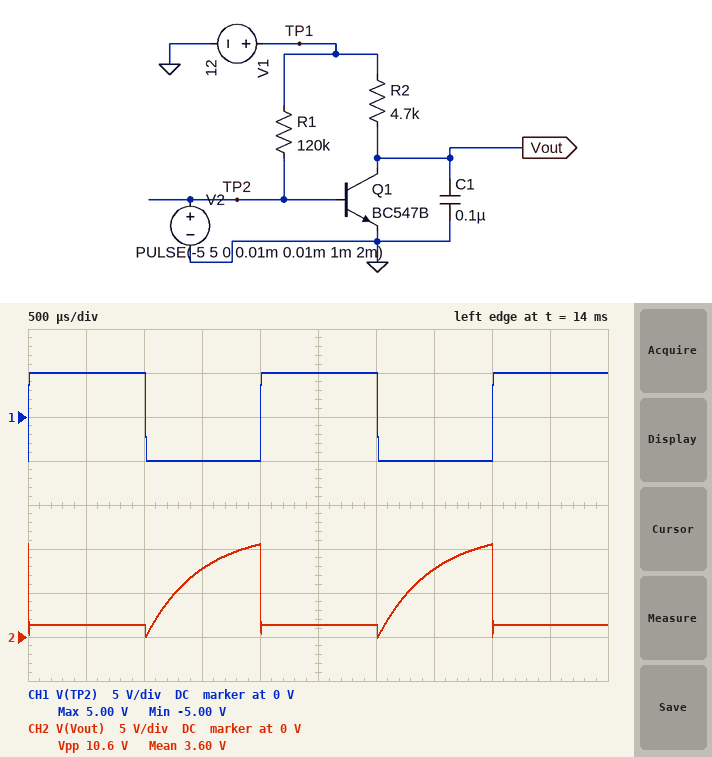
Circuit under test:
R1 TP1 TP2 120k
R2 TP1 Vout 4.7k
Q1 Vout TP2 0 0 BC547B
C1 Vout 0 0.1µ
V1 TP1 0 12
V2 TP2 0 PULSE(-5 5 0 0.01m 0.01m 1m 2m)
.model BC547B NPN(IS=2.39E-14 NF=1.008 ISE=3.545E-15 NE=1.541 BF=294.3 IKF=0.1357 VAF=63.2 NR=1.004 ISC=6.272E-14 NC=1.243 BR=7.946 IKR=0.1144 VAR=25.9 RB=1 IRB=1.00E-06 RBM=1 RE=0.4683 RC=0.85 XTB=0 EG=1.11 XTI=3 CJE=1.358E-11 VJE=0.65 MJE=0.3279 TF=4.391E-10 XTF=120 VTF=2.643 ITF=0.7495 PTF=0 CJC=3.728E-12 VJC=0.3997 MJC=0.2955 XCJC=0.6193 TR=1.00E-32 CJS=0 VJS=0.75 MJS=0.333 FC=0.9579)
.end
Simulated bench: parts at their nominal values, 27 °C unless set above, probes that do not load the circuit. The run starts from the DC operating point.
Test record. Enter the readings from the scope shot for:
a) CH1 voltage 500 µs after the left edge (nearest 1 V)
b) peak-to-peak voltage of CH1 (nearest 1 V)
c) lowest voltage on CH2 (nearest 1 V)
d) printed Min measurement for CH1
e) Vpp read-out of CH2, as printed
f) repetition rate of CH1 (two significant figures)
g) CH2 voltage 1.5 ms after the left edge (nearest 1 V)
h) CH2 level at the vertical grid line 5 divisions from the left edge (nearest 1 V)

5 V
10 V
0 V
-5.00 V
10.6 V
500 Hz
8 V
1 V
